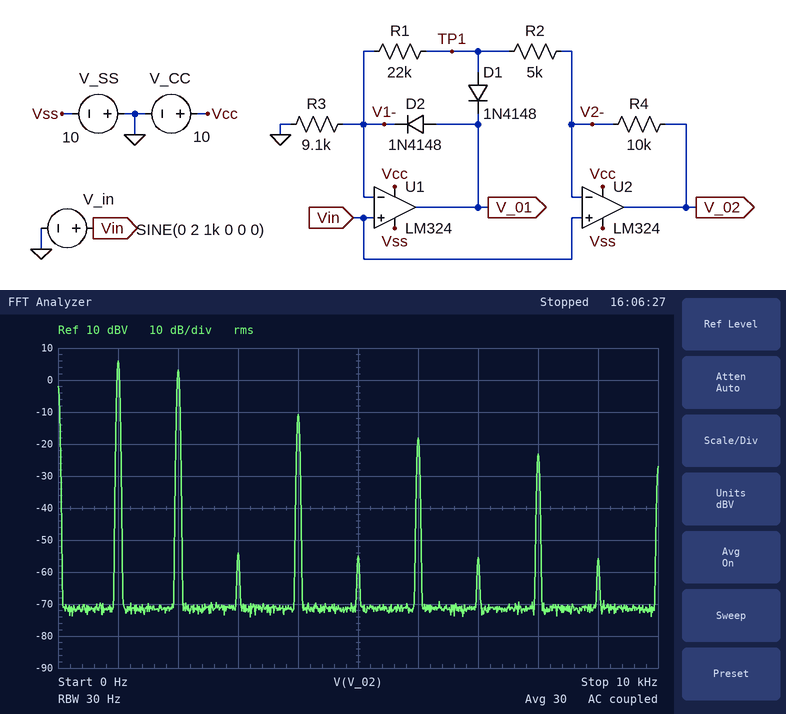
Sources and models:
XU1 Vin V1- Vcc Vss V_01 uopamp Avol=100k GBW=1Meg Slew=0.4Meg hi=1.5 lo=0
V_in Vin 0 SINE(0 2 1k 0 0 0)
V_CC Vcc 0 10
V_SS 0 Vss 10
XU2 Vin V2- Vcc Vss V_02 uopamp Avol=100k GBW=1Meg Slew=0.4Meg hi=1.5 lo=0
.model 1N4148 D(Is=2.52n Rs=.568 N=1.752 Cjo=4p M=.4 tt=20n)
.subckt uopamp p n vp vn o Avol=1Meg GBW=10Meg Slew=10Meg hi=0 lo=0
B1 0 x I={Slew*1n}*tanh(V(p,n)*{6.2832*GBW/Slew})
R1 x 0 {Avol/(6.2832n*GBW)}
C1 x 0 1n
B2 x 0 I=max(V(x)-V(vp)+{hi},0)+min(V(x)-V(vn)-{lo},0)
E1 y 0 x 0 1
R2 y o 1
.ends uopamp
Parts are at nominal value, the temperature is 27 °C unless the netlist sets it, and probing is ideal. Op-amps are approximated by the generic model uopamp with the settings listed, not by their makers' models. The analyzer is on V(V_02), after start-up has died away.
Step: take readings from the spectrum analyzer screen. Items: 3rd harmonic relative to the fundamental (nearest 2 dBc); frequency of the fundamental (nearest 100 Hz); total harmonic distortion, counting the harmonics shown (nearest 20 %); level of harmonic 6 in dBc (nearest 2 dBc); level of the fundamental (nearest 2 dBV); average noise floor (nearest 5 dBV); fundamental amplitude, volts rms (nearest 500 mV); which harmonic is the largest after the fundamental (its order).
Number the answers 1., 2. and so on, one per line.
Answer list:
1. -60 dBc
2. 1.0 kHz
3. 80 %
4. -24 dBc
5. 6 dBV
6. -70 dBV
7. 2.0 V
8. 2
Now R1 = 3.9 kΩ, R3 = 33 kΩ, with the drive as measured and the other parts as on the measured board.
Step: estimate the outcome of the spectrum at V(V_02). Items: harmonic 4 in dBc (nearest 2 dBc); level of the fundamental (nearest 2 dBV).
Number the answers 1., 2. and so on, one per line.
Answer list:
1. -38 dBc
2. 2 dBV
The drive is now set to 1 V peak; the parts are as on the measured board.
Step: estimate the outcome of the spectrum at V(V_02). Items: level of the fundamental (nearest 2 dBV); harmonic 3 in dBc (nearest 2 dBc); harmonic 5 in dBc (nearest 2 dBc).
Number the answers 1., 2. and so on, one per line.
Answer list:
1. 0 dBV
2. -56 dBc
3. -56 dBc
